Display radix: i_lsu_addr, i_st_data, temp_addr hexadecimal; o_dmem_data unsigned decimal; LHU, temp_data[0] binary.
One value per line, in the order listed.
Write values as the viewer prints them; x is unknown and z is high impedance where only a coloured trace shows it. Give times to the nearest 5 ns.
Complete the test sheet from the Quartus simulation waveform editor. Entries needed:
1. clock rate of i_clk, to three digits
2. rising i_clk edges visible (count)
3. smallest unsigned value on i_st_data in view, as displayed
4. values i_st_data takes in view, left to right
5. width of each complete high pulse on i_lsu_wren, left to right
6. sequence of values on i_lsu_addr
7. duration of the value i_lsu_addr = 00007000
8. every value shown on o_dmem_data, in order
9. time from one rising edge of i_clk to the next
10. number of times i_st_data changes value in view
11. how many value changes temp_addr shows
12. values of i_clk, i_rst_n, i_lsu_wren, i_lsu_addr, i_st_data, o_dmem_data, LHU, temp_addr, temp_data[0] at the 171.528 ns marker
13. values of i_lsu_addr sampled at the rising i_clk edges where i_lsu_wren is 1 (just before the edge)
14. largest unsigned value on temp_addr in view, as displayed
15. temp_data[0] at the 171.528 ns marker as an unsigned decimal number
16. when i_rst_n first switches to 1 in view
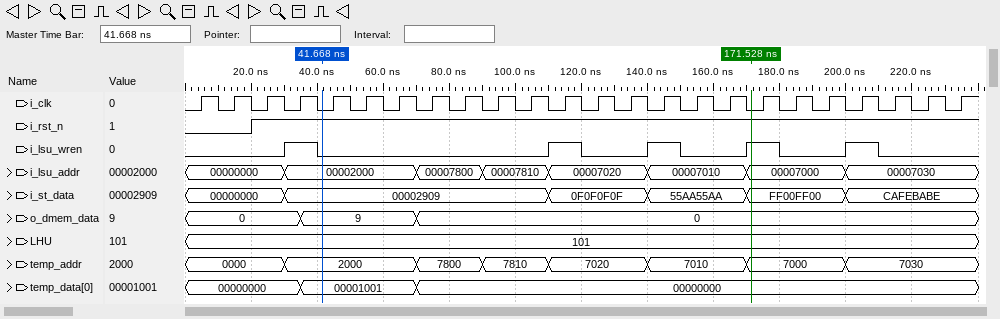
100 MHz
24
00000000
00000000, 00002909, 0F0F0F0F, 55AA55AA, FF00FF00, CAFEBABE
10 ns, 10 ns, 10 ns, 10 ns, 10 ns
00000000, 00002000, 00007800, 00007810, 00007020, 00007010, 00007000, 00007030
30 ns
0, 9, 0
10 ns
5
7
i_clk=0, i_rst_n=1, i_lsu_wren=1, i_lsu_addr=00007000, i_st_data=FF00FF00, o_dmem_data=0, LHU=101, temp_addr=7000, temp_data[0]=00000000
00002000, 00007020, 00007010, 00007000, 00007030
7810
0
20 ns
